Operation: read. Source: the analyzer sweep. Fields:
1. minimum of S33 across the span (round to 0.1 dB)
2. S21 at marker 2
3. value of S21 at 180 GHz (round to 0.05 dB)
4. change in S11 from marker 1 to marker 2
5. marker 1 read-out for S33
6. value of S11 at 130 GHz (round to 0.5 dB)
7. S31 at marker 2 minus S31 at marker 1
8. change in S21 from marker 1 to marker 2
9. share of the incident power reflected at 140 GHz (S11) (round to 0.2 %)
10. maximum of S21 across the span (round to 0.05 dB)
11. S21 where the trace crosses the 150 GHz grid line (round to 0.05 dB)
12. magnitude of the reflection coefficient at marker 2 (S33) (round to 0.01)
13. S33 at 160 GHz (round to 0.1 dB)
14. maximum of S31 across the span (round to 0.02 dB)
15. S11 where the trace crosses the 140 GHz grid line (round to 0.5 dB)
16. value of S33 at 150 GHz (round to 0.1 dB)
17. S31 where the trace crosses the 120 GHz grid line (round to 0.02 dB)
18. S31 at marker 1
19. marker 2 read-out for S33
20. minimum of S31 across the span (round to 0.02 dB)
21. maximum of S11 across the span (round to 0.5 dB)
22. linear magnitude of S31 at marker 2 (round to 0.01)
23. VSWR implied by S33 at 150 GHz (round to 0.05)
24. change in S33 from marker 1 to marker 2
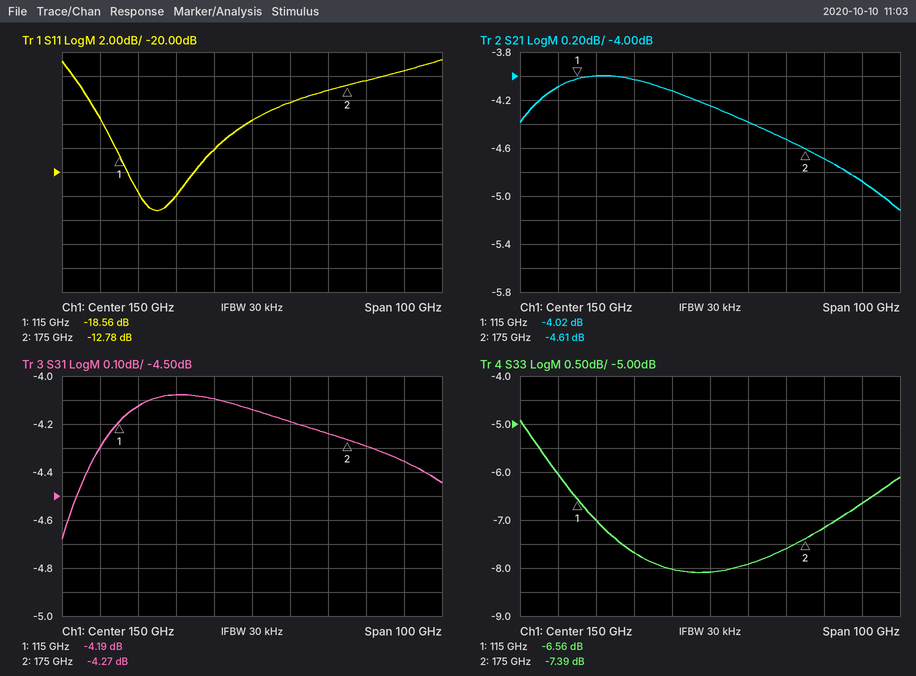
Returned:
-8.1 dB
-4.61 dB
-4.70 dB
5.78 dB
-6.56 dB
-22.0 dB
-0.08 dB
-0.59 dB
1.6 %
-4.00 dB
-4.25 dB
0.43
-7.9 dB
-4.08 dB
-18.0 dB
-8.1 dB
-4.12 dB
-4.19 dB
-7.39 dB
-4.68 dB
-10.5 dB
0.61
2.30
-0.83 dB
